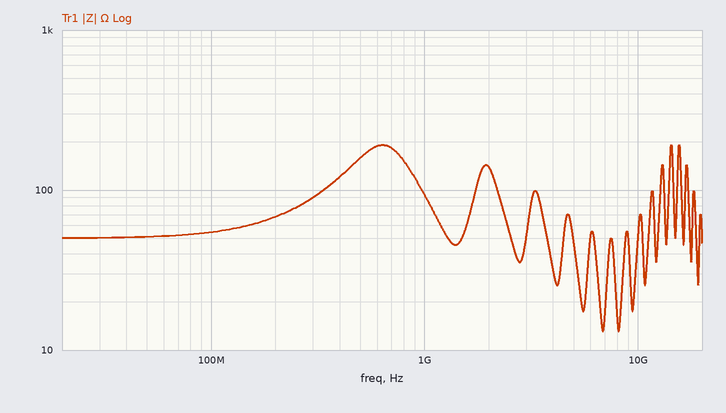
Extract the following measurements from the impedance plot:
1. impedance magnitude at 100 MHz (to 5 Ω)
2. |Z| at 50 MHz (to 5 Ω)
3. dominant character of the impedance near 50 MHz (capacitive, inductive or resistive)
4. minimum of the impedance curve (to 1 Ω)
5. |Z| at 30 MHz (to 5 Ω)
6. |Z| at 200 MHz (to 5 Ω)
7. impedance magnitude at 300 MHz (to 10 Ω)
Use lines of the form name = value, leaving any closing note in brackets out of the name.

impedance magnitude at 100 MHz = 55 Ω
|Z| at 50 MHz = 50 Ω
dominant character of the impedance near 50 MHz = resistive
minimum of the impedance curve = 13 Ω
|Z| at 30 MHz = 50 Ω
|Z| at 200 MHz = 70 Ω
impedance magnitude at 300 MHz = 90 Ω
